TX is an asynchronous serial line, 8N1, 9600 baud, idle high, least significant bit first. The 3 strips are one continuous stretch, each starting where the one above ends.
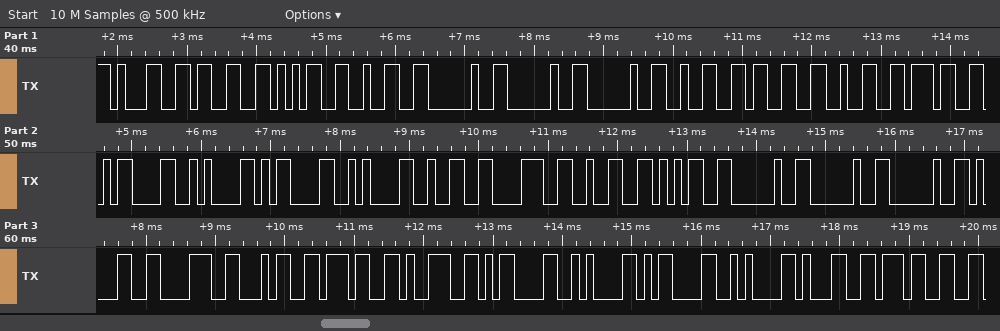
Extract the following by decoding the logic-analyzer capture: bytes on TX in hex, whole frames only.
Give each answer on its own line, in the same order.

0x31 0x33 0x35 0x32 0x20 0x20 0x20 0x32 0x33 0x32 0x37 0x0D 0x0A 0x0D 0x0A 0x32 0x38 0x32 0x35 0x20 0x20 0x20 0x31 0x38 0x34 0x37 0x39 0x0D 0x0A 0x0D 0x0A 0x31 0x37
